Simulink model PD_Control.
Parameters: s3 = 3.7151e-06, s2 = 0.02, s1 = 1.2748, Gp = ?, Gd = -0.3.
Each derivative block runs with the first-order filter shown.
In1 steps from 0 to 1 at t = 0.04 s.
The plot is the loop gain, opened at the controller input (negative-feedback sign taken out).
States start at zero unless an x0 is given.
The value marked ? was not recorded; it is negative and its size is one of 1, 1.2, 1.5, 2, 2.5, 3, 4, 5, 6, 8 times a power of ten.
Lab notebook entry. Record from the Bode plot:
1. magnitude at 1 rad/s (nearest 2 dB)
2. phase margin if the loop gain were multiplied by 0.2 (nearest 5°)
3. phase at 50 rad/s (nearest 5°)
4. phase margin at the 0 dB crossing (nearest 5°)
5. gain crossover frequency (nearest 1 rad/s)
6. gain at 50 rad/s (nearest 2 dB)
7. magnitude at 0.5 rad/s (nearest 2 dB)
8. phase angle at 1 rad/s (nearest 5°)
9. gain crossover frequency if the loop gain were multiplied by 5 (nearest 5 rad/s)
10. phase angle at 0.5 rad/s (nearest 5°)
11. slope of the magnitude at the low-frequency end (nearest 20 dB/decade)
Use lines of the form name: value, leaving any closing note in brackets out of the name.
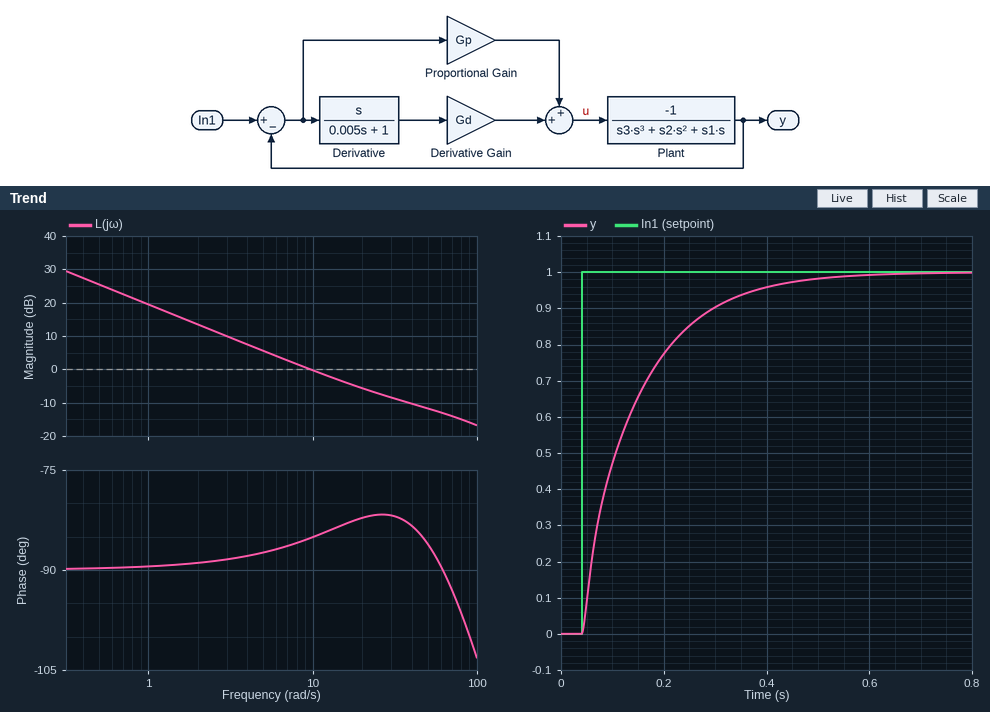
magnitude at 1 rad/s: 20 dB
phase margin if the loop gain were multiplied by 0.2: 90°
phase at 50 rad/s: -85°
phase margin at the 0 dB crossing: 95°
gain crossover frequency: 10 rad/s
gain at 50 rad/s: -12 dB
magnitude at 0.5 rad/s: 26 dB
phase angle at 1 rad/s: -90°
gain crossover frequency if the loop gain were multiplied by 5: 70 rad/s
phase angle at 0.5 rad/s: -90°
slope of the magnitude at the low-frequency end: -20 dB/decade
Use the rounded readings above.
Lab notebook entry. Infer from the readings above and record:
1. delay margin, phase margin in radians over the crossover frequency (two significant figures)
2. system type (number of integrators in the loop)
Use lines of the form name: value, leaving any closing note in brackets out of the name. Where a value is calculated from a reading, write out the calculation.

delay margin, phase margin in radians over the crossover frequency: 95 × π / 180 / 10 = 0.17 s
system type: 1
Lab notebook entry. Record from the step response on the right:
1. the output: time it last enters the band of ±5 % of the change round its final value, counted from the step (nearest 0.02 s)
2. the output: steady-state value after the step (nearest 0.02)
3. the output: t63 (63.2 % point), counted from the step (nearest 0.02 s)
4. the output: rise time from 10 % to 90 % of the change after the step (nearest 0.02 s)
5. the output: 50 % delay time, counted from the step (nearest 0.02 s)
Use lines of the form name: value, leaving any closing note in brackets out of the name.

the output: time it last enters the band of ±5 % of the change round its final value, counted from the step: 0.34 s
the output: steady-state value after the step: 1.00
the output: t63 (63.2 % point), counted from the step: 0.10 s
the output: rise time from 10 % to 90 % of the change after the step: 0.24 s
the output: 50 % delay time, counted from the step: 0.06 s
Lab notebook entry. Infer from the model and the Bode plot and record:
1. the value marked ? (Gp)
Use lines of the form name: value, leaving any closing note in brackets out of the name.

the value marked ?: -12
